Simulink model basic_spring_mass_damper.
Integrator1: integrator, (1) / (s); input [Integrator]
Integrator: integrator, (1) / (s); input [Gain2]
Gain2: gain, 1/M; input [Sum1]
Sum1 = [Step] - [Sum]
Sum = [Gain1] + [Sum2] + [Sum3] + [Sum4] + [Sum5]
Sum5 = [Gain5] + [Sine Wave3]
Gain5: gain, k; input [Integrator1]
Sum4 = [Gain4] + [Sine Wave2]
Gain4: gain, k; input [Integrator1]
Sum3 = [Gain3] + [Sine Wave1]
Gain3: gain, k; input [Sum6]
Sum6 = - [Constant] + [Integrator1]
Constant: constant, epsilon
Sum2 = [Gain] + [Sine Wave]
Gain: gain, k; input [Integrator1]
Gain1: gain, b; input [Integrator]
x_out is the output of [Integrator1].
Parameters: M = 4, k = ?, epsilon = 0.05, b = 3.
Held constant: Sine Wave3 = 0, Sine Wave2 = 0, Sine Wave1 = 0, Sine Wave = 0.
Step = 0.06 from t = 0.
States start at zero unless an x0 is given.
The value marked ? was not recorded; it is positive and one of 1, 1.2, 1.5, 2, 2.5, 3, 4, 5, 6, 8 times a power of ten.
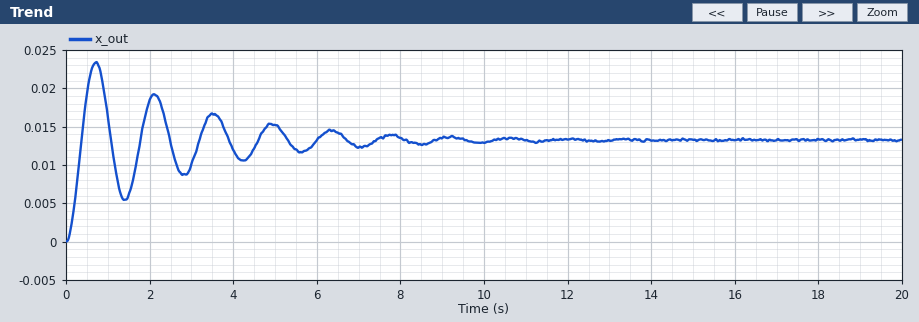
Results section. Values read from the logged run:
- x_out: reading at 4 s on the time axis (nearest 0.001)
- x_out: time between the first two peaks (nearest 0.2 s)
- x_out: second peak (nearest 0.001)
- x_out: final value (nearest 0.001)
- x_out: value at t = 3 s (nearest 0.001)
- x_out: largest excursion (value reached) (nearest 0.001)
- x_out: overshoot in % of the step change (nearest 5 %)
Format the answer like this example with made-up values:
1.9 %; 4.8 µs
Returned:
0.012; 1.4 s; 0.019; 0.013; 0.010; 0.023; 75 %
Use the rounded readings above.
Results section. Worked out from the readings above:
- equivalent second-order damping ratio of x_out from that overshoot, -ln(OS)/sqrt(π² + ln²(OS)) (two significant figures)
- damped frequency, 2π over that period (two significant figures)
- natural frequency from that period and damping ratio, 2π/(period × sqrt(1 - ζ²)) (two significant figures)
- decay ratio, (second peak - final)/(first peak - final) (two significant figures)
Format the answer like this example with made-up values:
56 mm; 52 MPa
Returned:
0.091; 4.5 rad/s; 4.5 rad/s; 0.60
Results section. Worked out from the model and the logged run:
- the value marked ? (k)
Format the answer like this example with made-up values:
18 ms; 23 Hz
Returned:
20
